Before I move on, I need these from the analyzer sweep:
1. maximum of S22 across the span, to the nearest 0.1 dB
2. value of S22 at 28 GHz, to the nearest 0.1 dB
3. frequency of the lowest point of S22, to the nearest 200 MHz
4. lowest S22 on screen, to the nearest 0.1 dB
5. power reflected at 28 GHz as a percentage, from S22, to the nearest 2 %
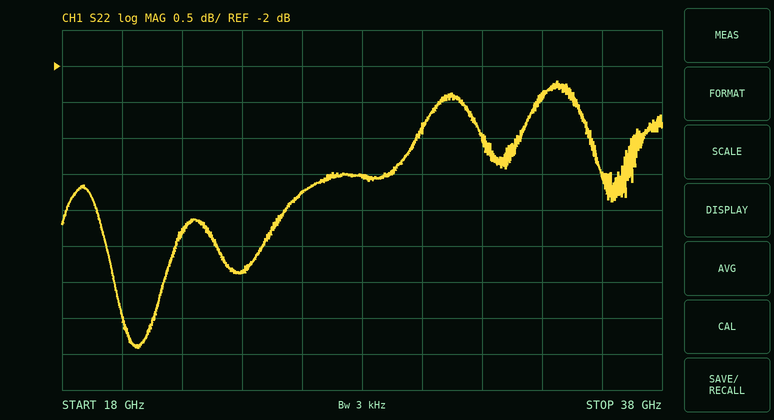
-2.2 dB
-3.5 dB
20.6 GHz
-5.9 dB
44 %
